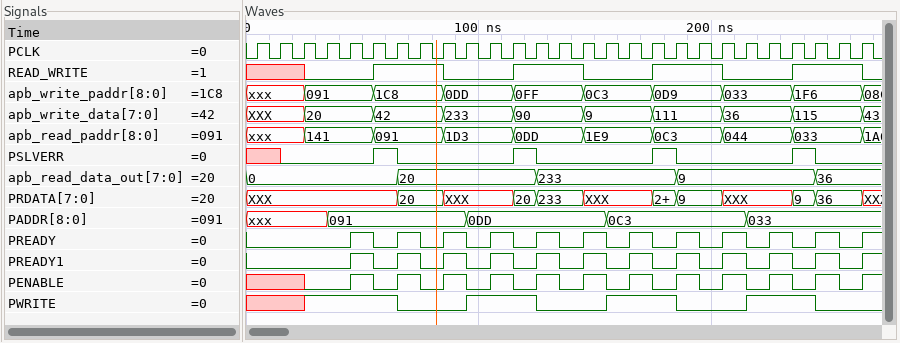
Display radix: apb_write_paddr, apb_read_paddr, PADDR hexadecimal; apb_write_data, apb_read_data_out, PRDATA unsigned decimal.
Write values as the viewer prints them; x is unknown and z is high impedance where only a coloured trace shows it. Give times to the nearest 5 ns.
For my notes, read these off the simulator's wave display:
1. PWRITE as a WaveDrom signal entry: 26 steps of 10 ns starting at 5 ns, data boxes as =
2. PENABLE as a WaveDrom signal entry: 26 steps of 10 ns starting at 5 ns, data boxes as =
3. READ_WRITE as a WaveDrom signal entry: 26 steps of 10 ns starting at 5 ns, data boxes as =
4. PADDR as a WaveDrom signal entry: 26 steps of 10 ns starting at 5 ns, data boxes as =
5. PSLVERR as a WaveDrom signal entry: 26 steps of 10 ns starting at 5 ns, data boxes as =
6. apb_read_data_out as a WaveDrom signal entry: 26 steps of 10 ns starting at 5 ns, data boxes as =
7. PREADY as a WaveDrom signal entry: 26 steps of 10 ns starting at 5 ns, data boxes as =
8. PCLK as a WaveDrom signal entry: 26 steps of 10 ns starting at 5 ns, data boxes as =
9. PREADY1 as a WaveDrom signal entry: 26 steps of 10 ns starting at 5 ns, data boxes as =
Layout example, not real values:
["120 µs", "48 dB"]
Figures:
["{name: 'PWRITE', wave: 'x.1...0..1..0..1..0..1..0.'}", "{name: 'PENABLE', wave: 'x.0.1010101010101010101010'}", "{name: 'READ_WRITE', wave: 'x.0..1..0..1..0..1..0..1..'}", "{name: 'PADDR', wave: 'x..=.....=.....=.....=....', data: '091 0DD 0C3 033'}", "{name: 'PSLVERR', wave: 'x0...10....10....10....10.'}", "{name: 'apb_read_data_out', wave: '=.....=.....=.....=.....=.', data: '0 20 233 9 36'}", "{name: 'PREADY', wave: '0...1010101010101010101010'}", "{name: 'PCLK', wave: 'p.........................'}", "{name: 'PREADY1', wave: '0...1010101010101010101010'}"]
